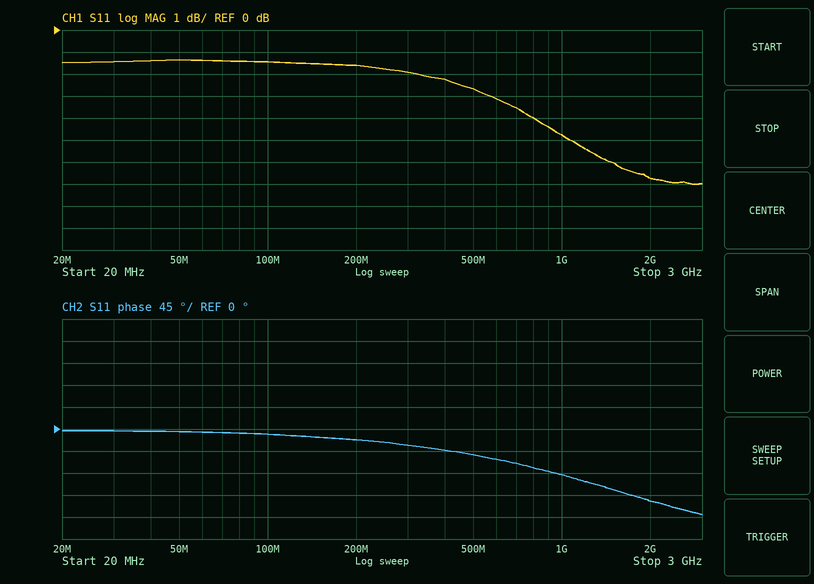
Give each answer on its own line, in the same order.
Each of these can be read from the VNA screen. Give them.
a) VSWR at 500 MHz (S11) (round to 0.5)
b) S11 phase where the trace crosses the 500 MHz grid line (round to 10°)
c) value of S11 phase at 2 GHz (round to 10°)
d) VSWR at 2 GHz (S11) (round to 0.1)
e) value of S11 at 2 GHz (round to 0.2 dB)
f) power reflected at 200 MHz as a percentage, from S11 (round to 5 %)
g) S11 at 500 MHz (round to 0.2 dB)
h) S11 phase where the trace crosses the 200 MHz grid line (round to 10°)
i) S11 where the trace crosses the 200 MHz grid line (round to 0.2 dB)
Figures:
6.5
-50°
-150°
2.7
-6.8 dB
70 %
-2.6 dB
-20°
-1.6 dB
